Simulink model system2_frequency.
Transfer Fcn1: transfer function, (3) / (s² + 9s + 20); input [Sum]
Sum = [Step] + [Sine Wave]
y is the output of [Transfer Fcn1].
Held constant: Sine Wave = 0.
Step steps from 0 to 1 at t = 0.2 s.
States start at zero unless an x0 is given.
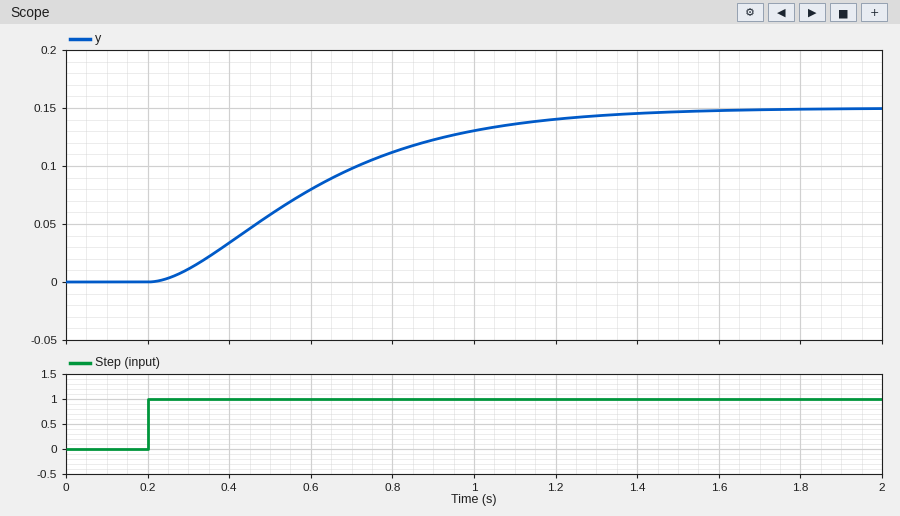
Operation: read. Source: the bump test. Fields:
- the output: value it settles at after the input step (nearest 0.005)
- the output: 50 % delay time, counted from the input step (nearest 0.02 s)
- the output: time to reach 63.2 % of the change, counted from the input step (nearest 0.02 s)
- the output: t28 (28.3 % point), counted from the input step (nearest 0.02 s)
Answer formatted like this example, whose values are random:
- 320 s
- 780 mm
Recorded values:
- 0.150
- 0.38 s
- 0.48 s
- 0.24 s
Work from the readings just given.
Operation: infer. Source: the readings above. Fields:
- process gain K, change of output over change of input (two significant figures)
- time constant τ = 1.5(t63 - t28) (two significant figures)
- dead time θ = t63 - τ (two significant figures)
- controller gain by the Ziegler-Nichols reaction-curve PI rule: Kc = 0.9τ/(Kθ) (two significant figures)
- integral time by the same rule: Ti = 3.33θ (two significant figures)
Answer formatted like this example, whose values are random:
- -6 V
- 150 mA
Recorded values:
- 0.15
- 0.36 s
- 0.12 s
- 18
- 0.40 s
